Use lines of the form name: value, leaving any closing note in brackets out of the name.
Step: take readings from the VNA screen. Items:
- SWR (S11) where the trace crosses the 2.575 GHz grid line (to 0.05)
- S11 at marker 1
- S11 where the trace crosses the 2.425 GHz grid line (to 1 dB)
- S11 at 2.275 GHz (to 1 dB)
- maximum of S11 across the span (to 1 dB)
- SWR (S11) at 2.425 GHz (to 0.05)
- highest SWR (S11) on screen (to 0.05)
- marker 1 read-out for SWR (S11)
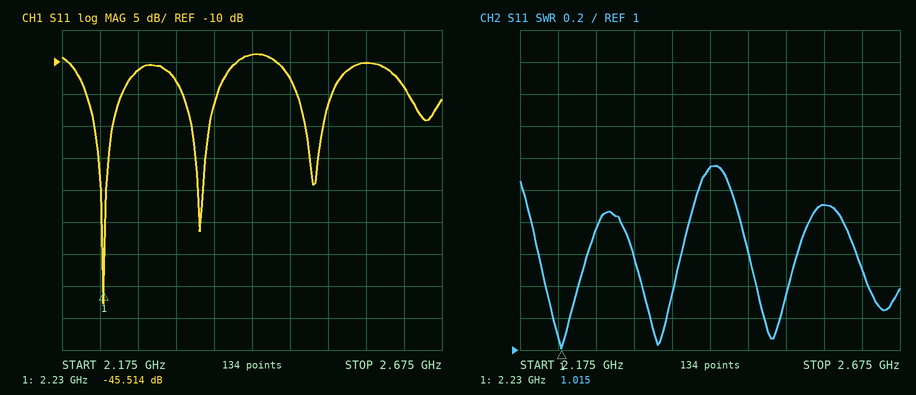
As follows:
SWR (S11) where the trace crosses the 2.575 GHz grid line: 1.90
S11 at marker 1: -45.514 dB
S11 where the trace crosses the 2.425 GHz grid line: -9 dB
S11 at 2.275 GHz: -11 dB
maximum of S11 across the span: -9 dB
SWR (S11) at 2.425 GHz: 2.15
highest SWR (S11) on screen: 2.15
marker 1 read-out for SWR: 1.015
